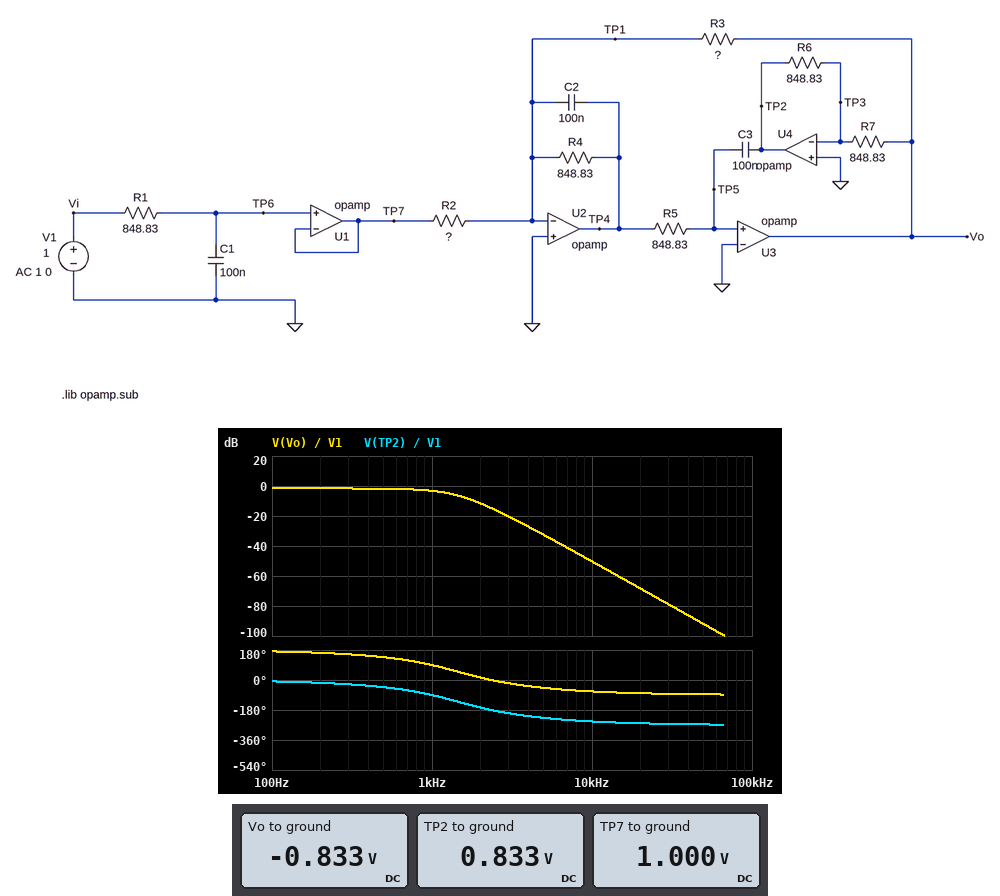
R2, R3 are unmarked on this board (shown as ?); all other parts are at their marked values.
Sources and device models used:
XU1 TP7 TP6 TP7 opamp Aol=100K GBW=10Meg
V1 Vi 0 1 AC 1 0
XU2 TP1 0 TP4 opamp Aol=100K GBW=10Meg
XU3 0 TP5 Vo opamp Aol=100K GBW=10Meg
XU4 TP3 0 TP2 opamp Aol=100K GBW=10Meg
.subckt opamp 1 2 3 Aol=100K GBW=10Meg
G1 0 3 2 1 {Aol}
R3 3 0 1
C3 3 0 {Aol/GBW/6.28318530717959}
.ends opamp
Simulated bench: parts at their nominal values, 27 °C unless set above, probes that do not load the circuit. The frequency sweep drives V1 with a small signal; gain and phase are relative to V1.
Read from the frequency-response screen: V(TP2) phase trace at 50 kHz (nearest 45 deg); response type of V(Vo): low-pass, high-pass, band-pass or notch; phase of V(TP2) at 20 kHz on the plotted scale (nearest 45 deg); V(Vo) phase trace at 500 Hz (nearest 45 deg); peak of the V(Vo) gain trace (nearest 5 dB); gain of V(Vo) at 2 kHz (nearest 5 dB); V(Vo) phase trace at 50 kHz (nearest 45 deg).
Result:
-270 deg
low-pass
-270 deg
135 deg
0 dB
-10 dB
-90 deg
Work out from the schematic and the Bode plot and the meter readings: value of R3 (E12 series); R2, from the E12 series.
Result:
1.5 kΩ
1.8 kΩ
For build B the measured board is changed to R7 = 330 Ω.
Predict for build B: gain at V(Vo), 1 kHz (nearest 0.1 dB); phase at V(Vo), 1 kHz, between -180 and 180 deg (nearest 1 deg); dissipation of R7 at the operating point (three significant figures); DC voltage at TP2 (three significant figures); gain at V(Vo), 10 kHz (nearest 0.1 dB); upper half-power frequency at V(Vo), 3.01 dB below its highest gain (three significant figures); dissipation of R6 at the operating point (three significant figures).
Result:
-10.4 dB
55 deg
2.10 mW
2.14 V
-58.6 dB
487 Hz
5.41 mW
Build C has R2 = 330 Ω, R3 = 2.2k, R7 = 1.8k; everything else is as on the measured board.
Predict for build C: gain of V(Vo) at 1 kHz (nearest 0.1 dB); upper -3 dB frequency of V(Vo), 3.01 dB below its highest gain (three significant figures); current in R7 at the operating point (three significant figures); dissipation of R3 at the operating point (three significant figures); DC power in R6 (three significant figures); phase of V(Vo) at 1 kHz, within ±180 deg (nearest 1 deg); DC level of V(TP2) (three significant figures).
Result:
16.1 dB
1.63 kHz
3.70 mA
20.2 mW
11.6 mW
107 deg
3.14 V
